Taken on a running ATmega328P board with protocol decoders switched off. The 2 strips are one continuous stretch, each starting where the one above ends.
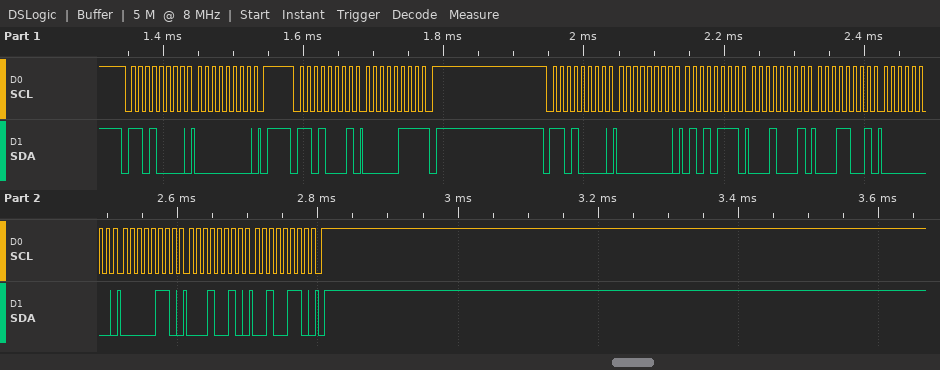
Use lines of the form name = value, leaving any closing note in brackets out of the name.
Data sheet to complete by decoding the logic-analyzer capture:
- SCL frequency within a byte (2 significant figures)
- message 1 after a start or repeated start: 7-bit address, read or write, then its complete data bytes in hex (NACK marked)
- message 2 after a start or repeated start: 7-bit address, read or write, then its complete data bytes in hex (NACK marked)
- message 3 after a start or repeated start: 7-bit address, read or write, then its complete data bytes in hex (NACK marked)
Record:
SCL frequency within a byte = 100 kHz
message 1 after a start or repeated start: 7-bit address, read or write, then its complete data bytes in hex = 0x68 write: 00
message 2 after a start or repeated start: 7-bit address, read or write, then its complete data bytes in hex = 0x68 read: 07 NACK
message 3 after a start or repeated start: 7-bit address, read or write, then its complete data bytes in hex = 0x68 write: 00 57 11 19 00 06 12 26
